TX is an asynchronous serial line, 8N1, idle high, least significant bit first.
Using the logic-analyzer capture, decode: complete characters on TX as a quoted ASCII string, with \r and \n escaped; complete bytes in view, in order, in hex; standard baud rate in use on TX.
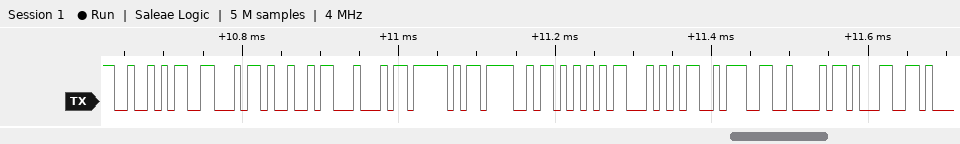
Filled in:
"RFID_OUT:B1"
52 46 49 44 5F 4F 55 54 3A 42 31
115200 baud
